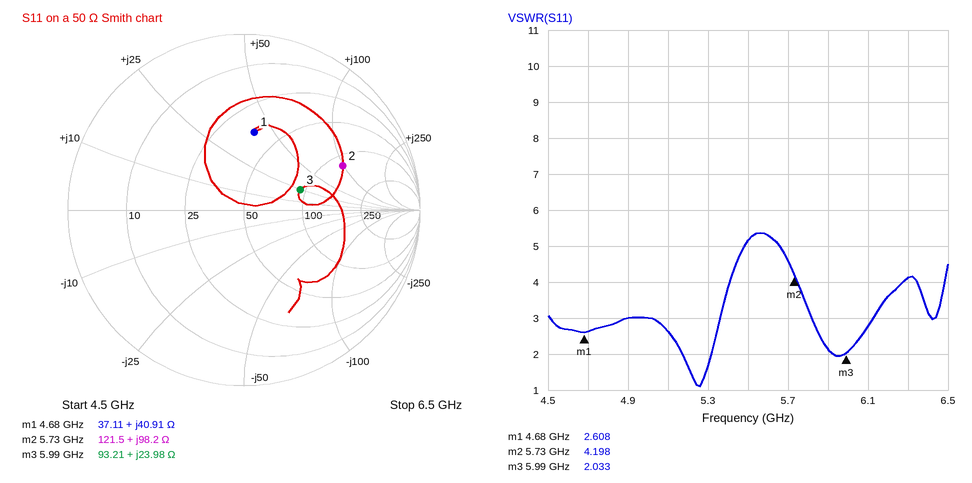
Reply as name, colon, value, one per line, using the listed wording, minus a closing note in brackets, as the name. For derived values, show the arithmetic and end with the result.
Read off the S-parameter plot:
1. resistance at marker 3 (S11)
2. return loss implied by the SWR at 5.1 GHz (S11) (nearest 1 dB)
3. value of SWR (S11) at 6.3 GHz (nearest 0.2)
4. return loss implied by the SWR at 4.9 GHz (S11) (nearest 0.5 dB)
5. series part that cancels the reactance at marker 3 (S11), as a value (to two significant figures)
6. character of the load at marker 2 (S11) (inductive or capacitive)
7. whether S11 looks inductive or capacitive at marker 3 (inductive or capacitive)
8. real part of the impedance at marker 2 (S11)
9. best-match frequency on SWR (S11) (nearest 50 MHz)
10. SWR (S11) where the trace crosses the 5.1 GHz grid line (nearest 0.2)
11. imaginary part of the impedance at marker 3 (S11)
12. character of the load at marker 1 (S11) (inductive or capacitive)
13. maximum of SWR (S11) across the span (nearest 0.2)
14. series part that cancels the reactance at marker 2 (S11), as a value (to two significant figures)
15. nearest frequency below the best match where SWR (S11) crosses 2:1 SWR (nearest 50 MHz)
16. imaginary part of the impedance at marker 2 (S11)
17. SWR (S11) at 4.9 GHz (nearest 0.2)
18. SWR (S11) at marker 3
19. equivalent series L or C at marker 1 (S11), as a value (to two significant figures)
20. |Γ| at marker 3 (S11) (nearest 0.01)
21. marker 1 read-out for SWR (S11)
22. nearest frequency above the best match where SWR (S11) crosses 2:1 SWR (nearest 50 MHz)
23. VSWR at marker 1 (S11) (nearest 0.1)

resistance at marker 3: 93.21 Ω
return loss implied by the SWR at 5.1 GHz (S11): −20 log10((2.6 − 1)/(2.6 + 1)) ≈ 7 dB
value of SWR (S11) at 6.3 GHz: 4.2
return loss implied by the SWR at 4.9 GHz (S11): −20 log10((3 − 1)/(3 + 1)) ≈ 6.0 dB
series part that cancels the reactance at marker 3 (S11), as a value: C = 1/(2π × 5.99 GHz × 23.98 Ω) ≈ 1.1 pF
character of the load at marker 2 (S11): inductive
whether S11 looks inductive or capacitive at marker 3: inductive
real part of the impedance at marker 2: 121.5 Ω
best-match frequency on SWR (S11): 5.25 GHz
SWR (S11) where the trace crosses the 5.1 GHz grid line: 2.6
imaginary part of the impedance at marker 3: +23.98 Ω
character of the load at marker 1 (S11): inductive
maximum of SWR (S11) across the span: 5.4
series part that cancels the reactance at marker 2 (S11), as a value: C = 1/(2π × 5.73 GHz × 98.2 Ω) ≈ 283 fF, so 280 fF to two significant figures
nearest frequency below the best match where SWR (S11) crosses 2:1 SWR: 5.15 GHz
imaginary part of the impedance at marker 2: +98.2 Ω
SWR (S11) at 4.9 GHz: 3.0
SWR (S11) at marker 3: 2.033
equivalent series L or C at marker 1 (S11), as a value: L = 40.91 Ω/(2π × 4.68 GHz) ≈ 1.4 nH
|Γ| at marker 3 (S11): 0.34
marker 1 read-out for SWR: 2.608
nearest frequency above the best match where SWR (S11) crosses 2:1 SWR: 5.30 GHz
VSWR at marker 1 (S11): 2.6
